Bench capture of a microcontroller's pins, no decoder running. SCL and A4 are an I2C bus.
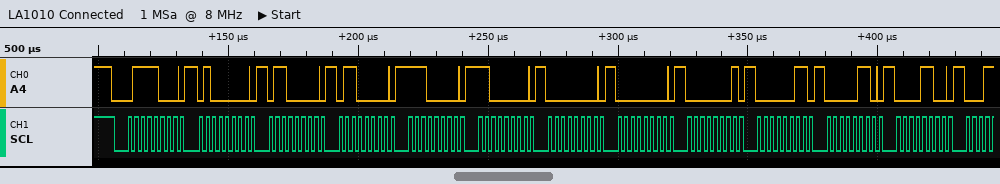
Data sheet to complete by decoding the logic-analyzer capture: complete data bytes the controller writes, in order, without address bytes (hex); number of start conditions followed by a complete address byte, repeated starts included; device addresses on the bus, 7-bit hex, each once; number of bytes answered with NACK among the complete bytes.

40 60 60 E0 C0 00 00 01 03 06 0C
1
0x3C
0
